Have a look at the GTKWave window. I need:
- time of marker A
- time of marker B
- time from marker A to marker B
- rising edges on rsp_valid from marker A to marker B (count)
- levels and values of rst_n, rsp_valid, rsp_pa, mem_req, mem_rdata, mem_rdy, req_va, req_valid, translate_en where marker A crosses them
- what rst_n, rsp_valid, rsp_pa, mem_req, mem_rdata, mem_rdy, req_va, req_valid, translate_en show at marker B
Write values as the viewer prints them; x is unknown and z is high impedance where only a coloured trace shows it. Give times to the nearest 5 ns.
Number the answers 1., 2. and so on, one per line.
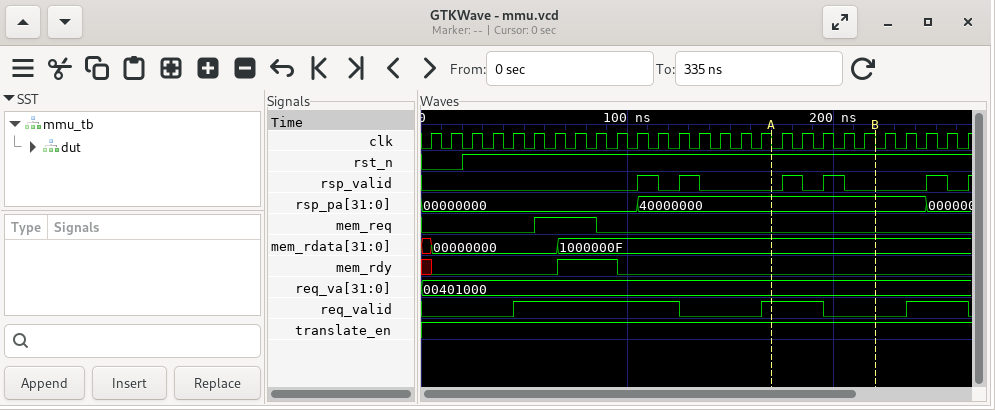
1. 170 ns
2. 220 ns
3. 50 ns
4. 2
5. rst_n=1, rsp_valid=0, rsp_pa=40000000, mem_req=0, mem_rdata=1000000F, mem_rdy=0, req_va=00401000, req_valid=1, translate_en=1
6. rst_n=1, rsp_valid=0, rsp_pa=40000000, mem_req=0, mem_rdata=1000000F, mem_rdy=0, req_va=00401000, req_valid=0, translate_en=1
